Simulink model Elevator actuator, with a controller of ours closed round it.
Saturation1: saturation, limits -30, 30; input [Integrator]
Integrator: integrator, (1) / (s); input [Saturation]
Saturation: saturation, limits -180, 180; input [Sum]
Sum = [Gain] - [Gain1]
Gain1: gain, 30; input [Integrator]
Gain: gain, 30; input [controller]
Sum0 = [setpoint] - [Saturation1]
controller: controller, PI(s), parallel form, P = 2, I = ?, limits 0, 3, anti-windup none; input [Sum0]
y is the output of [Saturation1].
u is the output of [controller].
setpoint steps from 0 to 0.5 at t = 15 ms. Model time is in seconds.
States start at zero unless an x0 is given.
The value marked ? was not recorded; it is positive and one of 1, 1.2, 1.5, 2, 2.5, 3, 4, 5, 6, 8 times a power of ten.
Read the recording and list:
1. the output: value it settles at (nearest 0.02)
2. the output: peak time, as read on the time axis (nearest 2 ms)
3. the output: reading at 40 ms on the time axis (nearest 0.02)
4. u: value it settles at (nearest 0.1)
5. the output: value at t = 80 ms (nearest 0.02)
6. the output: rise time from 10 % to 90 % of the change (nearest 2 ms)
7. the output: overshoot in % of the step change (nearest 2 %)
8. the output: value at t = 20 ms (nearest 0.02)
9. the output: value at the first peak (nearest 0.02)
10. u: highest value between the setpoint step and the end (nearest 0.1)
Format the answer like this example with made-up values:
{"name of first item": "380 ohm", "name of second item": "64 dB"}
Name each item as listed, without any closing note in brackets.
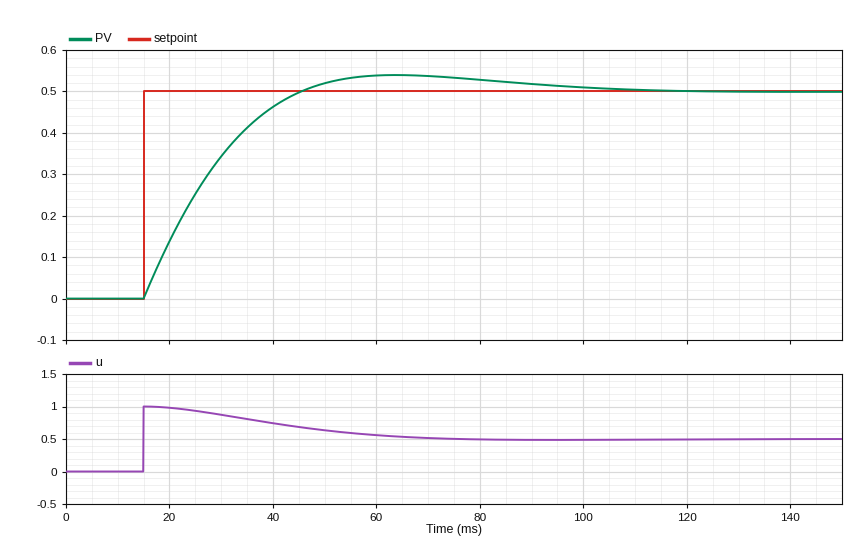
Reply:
{"the output: value it settles at": "0.50", "the output: peak time, as read on the time axis": "64 ms", "the output: reading at 40 ms on the time axis": "0.46", "u: value it settles at": "0.5", "the output: value at t = 80 ms": "0.52", "the output: rise time from 10 % to 90 % of the change": "22 ms", "the output: overshoot in % of the step change": "8 %", "the output: value at t = 20 ms": "0.14", "the output: value at the first peak": "0.54", "u: highest value between the setpoint step and the end": "1.0"}
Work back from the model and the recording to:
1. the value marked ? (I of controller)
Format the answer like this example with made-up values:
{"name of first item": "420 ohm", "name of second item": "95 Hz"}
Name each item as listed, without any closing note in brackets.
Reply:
{"the value marked ?": "120"}
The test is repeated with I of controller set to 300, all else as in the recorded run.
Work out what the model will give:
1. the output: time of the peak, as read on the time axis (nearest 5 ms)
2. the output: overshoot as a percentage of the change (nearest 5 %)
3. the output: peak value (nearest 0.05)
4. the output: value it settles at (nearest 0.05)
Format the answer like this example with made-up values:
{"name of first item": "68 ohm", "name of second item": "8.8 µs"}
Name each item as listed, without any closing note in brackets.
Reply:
{"the output: time of the peak, as read on the time axis": "45 ms", "the output: overshoot as a percentage of the change": "25 %", "the output: peak value": "0.60", "the output: value it settles at": "0.50"}
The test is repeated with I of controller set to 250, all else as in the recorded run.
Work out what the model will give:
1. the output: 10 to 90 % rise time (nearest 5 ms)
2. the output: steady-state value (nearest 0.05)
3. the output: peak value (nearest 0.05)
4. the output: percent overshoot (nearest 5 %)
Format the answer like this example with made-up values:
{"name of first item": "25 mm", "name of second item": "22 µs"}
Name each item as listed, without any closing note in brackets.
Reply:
{"the output: 10 to 90 % rise time": "15 ms", "the output: steady-state value": "0.50", "the output: peak value": "0.60", "the output: percent overshoot": "20 %"}
